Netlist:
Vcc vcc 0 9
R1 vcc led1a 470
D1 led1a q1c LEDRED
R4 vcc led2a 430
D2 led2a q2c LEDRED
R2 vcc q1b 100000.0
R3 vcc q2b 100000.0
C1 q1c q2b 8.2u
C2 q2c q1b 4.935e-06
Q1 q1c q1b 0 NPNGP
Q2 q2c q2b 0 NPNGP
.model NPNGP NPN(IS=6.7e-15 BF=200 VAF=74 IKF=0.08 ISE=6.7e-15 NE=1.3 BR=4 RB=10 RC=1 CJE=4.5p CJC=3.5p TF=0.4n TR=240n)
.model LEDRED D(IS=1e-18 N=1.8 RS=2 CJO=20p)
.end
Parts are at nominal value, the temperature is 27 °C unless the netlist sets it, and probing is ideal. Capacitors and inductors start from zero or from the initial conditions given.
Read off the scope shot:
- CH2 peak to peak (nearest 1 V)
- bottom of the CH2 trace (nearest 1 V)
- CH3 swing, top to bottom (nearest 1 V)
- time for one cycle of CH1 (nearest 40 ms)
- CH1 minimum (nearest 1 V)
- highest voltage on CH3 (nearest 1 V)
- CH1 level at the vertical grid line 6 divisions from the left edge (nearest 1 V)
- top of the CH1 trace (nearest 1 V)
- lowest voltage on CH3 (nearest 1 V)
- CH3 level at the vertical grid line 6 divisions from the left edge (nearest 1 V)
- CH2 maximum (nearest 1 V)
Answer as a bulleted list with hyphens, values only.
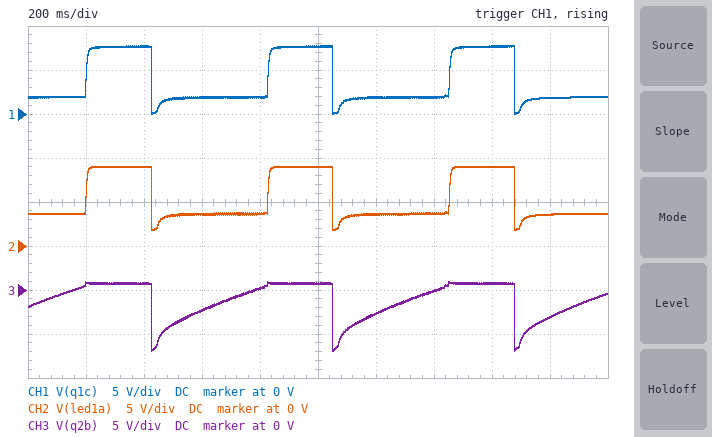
- 7 V
- 2 V
- 8 V
- 640 ms
- 0 V
- 1 V
- 2 V
- 8 V
- -7 V
- -3 V
- 9 V
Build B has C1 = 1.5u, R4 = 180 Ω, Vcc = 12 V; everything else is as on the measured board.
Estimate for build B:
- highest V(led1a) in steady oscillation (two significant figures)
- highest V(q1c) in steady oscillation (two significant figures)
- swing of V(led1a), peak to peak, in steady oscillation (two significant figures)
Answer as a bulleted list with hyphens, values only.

- 12 V
- 11 V
- 10 V
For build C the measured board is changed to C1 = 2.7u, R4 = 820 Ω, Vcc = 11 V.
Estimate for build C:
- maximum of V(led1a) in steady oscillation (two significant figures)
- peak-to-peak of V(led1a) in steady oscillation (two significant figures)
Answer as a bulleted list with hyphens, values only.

- 11 V
- 9.2 V
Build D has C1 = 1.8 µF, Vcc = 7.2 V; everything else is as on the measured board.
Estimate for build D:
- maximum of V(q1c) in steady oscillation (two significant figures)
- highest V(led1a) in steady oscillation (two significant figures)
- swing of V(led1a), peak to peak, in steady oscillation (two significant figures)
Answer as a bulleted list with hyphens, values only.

- 6.0 V
- 7.2 V
- 5.4 V
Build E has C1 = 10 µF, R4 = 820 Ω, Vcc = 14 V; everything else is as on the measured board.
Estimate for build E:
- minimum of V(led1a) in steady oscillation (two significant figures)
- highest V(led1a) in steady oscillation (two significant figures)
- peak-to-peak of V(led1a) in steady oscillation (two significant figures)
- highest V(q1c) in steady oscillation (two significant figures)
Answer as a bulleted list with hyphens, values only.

- 1.9 V
- 14 V
- 12 V
- 13 V
